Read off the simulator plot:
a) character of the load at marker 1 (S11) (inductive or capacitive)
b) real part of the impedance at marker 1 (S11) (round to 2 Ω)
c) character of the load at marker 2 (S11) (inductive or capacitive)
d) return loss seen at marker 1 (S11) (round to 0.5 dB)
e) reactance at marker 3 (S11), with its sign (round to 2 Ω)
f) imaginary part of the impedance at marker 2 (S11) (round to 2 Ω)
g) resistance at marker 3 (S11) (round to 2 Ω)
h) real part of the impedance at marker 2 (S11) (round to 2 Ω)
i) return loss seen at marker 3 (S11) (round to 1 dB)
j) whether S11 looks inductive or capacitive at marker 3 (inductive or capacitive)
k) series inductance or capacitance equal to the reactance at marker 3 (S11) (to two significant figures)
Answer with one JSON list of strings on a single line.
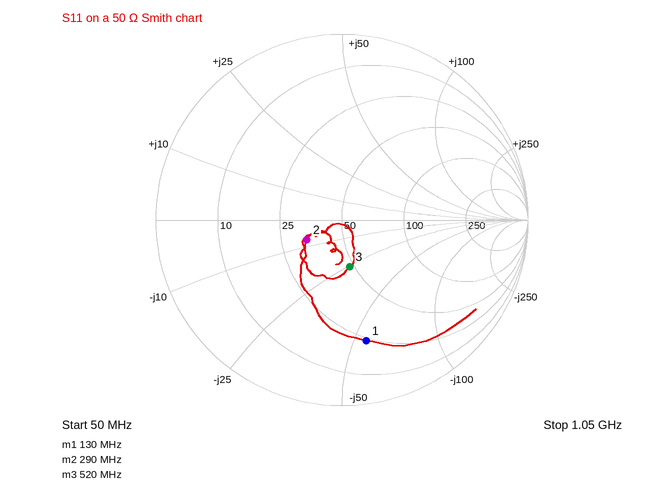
["capacitive", "24 Ω", "capacitive", "3.5 dB", "-26 Ω", "-8 Ω", "48 Ω", "34 Ω", "12 dB", "capacitive", "12 pF"]
